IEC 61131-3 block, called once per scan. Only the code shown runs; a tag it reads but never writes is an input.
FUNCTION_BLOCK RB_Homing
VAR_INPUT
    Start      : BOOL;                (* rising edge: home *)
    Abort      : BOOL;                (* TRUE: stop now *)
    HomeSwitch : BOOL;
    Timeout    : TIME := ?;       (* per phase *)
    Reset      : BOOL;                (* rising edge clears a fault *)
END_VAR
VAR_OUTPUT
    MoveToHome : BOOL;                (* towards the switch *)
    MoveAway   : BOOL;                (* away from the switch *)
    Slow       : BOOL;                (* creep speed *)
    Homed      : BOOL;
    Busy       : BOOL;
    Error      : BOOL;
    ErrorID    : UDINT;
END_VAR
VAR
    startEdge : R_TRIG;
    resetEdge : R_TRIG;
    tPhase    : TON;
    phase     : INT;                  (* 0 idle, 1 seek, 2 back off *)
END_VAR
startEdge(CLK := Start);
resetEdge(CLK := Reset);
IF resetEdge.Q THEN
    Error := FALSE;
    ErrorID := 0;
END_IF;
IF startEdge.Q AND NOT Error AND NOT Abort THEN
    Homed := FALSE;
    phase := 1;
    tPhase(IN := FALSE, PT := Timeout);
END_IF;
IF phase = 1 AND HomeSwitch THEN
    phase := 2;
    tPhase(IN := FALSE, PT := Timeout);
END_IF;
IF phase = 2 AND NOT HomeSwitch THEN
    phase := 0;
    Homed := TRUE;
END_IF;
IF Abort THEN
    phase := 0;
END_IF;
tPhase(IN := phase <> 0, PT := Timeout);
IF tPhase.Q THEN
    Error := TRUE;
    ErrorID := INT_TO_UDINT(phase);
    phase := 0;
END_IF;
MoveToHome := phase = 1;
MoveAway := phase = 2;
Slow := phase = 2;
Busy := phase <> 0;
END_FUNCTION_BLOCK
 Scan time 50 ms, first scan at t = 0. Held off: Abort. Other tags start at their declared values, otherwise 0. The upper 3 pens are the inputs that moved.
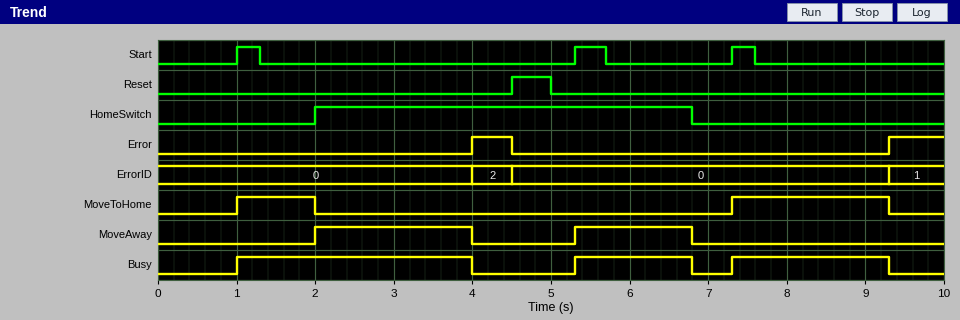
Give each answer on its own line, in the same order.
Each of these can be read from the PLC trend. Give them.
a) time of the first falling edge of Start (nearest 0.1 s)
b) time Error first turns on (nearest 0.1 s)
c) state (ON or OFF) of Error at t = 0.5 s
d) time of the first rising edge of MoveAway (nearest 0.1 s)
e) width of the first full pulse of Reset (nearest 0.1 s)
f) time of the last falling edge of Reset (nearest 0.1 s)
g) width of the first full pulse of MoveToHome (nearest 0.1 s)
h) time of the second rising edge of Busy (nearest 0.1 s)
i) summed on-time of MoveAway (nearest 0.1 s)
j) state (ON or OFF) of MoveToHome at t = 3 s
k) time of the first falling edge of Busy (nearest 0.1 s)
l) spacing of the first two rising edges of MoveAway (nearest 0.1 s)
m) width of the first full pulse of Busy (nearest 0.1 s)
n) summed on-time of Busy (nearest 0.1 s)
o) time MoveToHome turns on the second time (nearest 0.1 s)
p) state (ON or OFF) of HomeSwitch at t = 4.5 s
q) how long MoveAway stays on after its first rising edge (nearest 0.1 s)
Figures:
1.3 s
4.0 s
OFF
2.0 s
0.5 s
5.0 s
1.0 s
5.3 s
3.5 s
OFF
4.0 s
3.3 s
3.0 s
6.5 s
7.3 s
ON
2.0 s
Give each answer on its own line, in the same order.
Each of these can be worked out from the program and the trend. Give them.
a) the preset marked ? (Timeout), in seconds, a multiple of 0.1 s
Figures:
2.0 s
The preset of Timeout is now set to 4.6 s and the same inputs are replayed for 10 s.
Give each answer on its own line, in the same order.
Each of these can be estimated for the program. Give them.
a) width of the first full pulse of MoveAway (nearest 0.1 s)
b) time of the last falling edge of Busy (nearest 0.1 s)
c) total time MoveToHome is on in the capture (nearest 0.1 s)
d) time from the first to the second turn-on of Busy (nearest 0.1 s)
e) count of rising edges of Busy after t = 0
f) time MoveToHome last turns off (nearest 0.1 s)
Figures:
4.8 s
6.8 s
3.7 s
6.3 s
2
2.0 s
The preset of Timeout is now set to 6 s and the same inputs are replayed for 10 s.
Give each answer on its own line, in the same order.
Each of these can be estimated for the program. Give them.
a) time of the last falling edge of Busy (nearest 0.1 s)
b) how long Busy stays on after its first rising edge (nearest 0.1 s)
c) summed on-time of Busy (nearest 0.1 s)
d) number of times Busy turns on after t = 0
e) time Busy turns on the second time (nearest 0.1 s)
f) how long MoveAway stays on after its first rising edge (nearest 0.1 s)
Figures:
6.8 s
5.8 s
8.5 s
2
7.3 s
4.8 s
